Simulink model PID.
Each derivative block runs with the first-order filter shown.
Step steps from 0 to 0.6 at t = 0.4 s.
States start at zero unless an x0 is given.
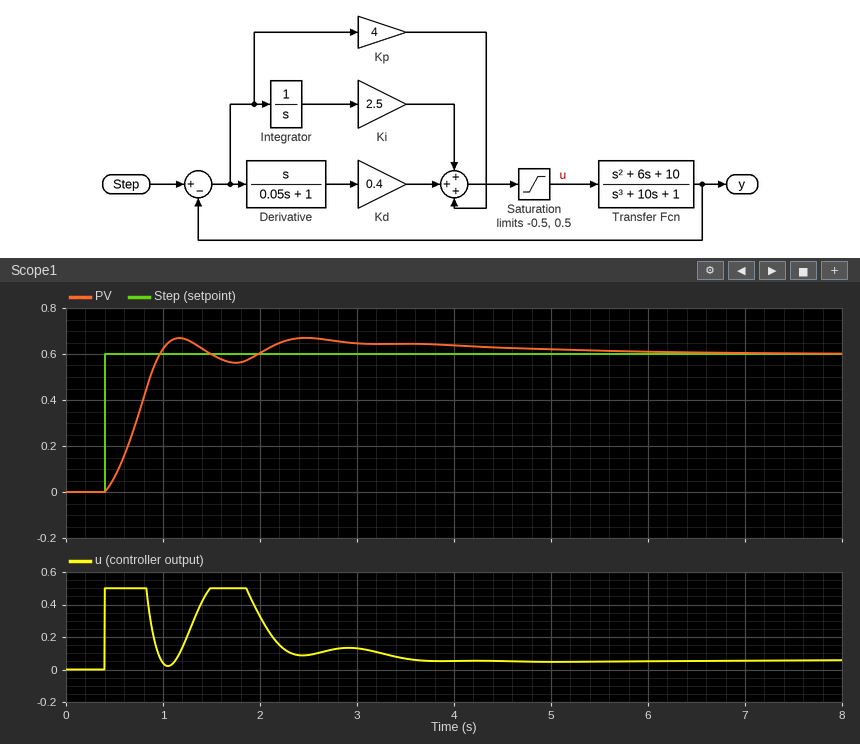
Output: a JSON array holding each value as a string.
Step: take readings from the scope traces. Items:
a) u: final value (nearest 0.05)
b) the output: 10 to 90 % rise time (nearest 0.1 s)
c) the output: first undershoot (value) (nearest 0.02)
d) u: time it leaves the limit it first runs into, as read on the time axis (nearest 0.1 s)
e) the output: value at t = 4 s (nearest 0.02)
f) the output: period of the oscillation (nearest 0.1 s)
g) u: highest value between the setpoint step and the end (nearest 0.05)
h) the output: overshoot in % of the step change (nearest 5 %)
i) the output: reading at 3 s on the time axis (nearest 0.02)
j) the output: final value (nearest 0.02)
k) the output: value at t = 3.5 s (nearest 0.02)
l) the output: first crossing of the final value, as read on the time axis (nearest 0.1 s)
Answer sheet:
["0.05", "0.4 s", "0.56", "0.8 s", "0.64", "1.3 s", "0.50", "10 %", "0.64", "0.60", "0.64", "1.0 s"]
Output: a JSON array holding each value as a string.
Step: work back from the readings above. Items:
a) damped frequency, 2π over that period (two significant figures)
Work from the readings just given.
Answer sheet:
["4.8 rad/s"]
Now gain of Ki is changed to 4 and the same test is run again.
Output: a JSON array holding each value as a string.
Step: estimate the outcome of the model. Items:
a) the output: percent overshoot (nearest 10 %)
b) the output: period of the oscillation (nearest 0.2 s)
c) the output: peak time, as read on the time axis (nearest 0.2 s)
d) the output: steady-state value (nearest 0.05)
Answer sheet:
["20 %", "1.2 s", "1.2 s", "0.60"]
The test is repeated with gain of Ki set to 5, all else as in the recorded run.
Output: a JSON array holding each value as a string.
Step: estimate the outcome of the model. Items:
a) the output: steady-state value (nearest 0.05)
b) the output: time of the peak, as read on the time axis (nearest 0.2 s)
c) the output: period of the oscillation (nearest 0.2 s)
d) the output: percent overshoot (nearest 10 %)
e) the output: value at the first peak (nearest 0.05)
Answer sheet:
["0.60", "1.2 s", "1.2 s", "30 %", "0.75"]
